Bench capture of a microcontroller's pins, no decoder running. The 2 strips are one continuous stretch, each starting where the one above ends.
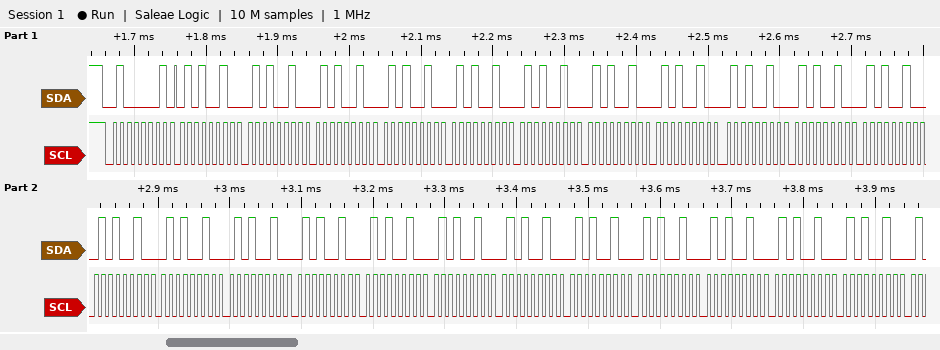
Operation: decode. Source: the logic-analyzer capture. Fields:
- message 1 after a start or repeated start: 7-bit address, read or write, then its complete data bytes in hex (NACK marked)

0x20 read: 52 52 52 52 52 52 52 52 52 52 52 52 52 52 52 52 52 52 52 52 52 52 52
